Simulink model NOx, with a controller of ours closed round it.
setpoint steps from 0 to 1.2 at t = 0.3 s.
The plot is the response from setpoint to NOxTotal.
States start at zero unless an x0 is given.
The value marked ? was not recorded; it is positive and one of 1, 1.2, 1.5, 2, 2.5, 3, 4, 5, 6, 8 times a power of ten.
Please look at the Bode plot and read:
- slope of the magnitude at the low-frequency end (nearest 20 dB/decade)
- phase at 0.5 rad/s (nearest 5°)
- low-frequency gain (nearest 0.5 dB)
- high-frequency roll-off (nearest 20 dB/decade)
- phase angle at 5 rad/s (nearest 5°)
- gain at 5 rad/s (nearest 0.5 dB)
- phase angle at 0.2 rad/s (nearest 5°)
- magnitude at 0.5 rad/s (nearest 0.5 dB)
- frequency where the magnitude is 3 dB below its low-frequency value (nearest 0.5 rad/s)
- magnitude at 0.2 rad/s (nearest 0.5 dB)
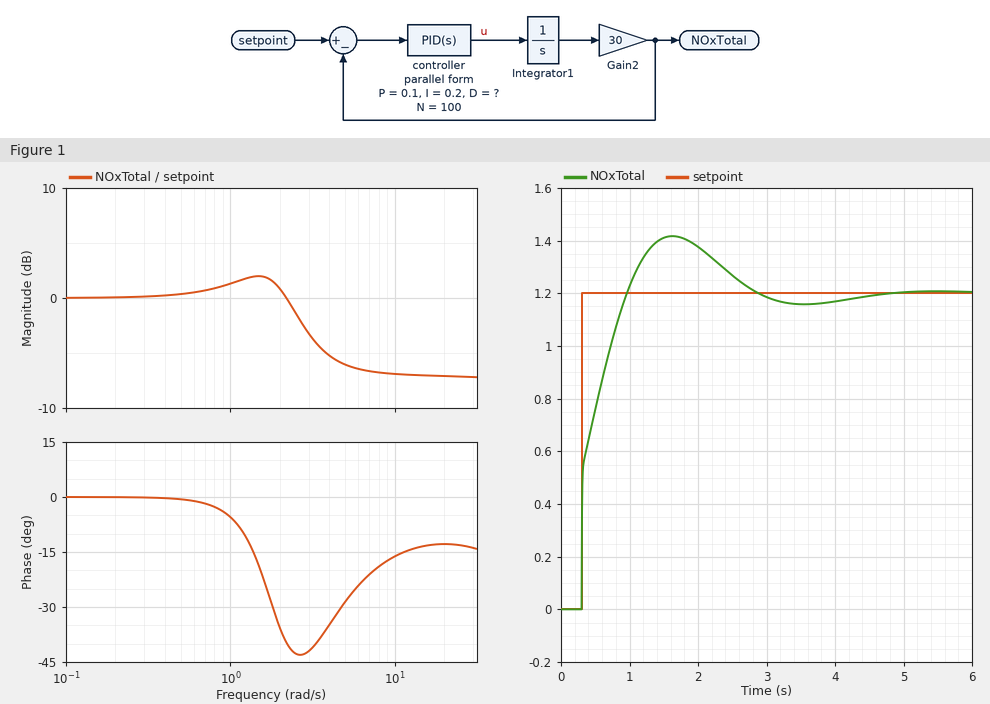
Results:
0 dB/decade
0°
0.0 dB
0 dB/decade
-30°
-6.0 dB
0°
0.5 dB
3.0 rad/s
0.0 dB
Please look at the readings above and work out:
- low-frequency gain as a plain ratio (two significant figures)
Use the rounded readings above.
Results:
1.0
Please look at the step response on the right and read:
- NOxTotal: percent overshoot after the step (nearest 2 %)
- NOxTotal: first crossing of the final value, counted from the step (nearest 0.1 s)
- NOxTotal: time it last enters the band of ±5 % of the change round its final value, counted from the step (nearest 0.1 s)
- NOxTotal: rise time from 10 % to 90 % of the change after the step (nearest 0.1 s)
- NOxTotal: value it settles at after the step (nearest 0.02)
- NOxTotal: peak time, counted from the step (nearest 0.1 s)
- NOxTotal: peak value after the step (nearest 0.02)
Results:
18 %
0.7 s
2.2 s
0.5 s
1.20
1.3 s
1.42
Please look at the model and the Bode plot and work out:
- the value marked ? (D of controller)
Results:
0.025
